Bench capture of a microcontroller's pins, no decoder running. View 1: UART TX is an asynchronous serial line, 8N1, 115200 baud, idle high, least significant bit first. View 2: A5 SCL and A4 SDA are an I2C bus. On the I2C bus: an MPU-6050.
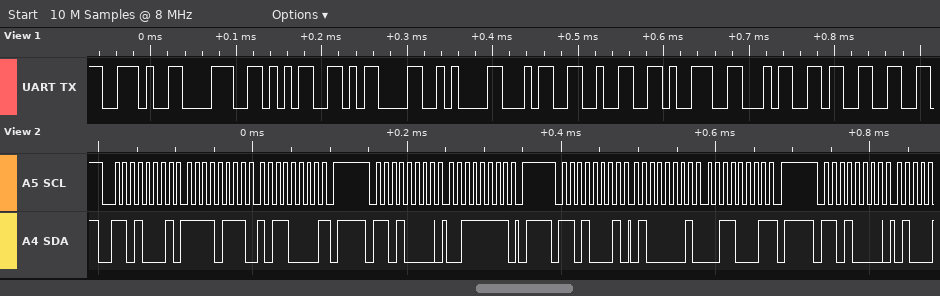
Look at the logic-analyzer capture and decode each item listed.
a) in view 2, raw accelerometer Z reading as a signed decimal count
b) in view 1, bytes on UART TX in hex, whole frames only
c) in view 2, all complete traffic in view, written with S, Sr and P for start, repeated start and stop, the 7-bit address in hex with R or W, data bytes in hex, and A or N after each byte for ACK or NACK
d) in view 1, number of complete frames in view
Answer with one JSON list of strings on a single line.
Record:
["16689", "2E 38 35 0D 0A 34 32 39 34 33", "S 68R A F7 A B0 N P S 68W A 3F A P S 68R A 41 A 31 N P S 68W A", "10"]
